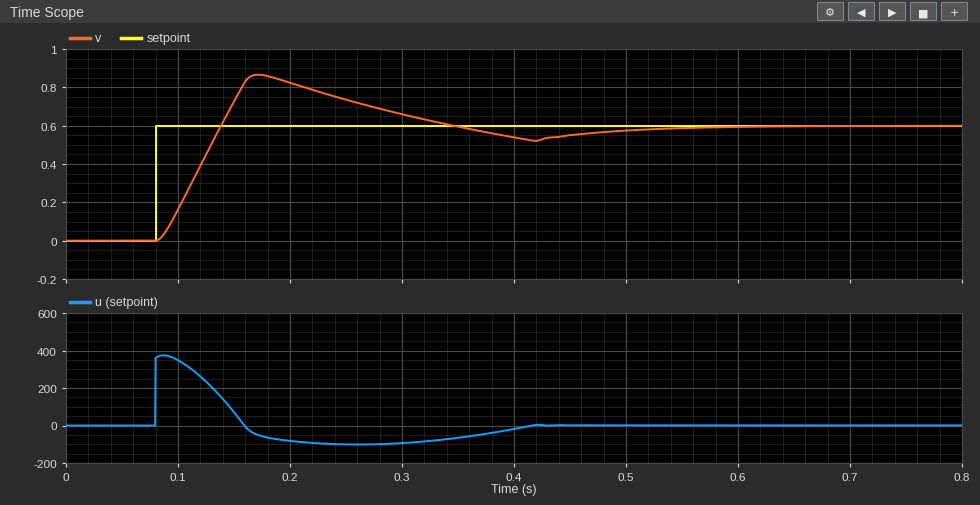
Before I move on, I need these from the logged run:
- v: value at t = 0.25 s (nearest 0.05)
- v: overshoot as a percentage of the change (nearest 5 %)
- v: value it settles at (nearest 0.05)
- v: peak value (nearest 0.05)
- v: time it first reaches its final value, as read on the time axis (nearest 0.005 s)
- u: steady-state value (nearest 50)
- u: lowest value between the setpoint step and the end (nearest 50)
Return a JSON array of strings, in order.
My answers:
["0.75", "45 %", "0.60", "0.85", "0.140 s", "0", "-100"]
